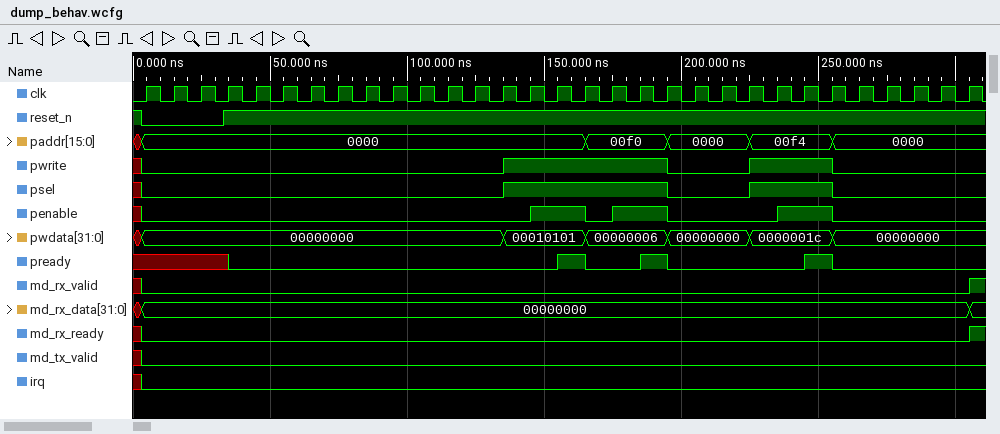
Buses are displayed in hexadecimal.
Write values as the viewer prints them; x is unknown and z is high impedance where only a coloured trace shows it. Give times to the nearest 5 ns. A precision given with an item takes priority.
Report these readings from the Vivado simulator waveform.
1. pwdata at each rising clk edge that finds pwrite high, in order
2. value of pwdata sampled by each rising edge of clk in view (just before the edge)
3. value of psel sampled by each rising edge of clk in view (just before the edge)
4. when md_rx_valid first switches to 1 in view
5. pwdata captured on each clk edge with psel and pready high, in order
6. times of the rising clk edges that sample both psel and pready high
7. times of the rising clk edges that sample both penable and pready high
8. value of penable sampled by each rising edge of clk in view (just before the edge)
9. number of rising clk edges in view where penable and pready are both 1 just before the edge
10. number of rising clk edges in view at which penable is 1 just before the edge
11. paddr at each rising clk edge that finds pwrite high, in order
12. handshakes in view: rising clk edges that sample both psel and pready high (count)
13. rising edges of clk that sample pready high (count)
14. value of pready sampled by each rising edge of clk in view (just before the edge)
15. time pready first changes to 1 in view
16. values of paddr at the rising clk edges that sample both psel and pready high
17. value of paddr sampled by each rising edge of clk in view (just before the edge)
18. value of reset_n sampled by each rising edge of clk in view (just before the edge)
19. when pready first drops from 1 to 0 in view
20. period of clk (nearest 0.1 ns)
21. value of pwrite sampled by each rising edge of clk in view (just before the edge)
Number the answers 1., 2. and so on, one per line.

1. 00010101, 00010101, 00010101, 00000006, 00000006, 00000006, 0000001c, 0000001c, 0000001c
2. 00000000, 00000000, 00000000, 00000000, 00000000, 00000000, 00000000, 00000000, 00000000, 00000000, 00000000, 00000000, 00000000, 00000000, 00010101, 00010101, 00010101, 00000006, 00000006, 00000006, 00000000, 00000000, 00000000, 0000001c, 0000001c, 0000001c, 00000000, 00000000, 00000000, 00000000, 00000000
3. 0 0 0 0 0 0 0 0 0 0 0 0 0 0 1 1 1 1 1 1 0 0 0 1 1 1 0 0 0 0 0
4. 305 ns
5. 00010101, 00000006, 0000001c
6. 165 ns, 195 ns, 255 ns
7. 165 ns, 195 ns, 255 ns
8. 0 0 0 0 0 0 0 0 0 0 0 0 0 0 0 1 1 0 1 1 0 0 0 0 1 1 0 0 0 0 0
9. 3
10. 6
11. 0000, 0000, 0000, 00f0, 00f0, 00f0, 00f4, 00f4, 00f4
12. 3
13. 3
14. x x x x 0 0 0 0 0 0 0 0 0 0 0 0 1 0 0 1 0 0 0 0 0 1 0 0 0 0 0
15. 155 ns
16. 0000, 00f0, 00f4
17. 0000, 0000, 0000, 0000, 0000, 0000, 0000, 0000, 0000, 0000, 0000, 0000, 0000, 0000, 0000, 0000, 0000, 00f0, 00f0, 00f0, 0000, 0000, 0000, 00f4, 00f4, 00f4, 0000, 0000, 0000, 0000, 0000
18. 0 0 0 1 1 1 1 1 1 1 1 1 1 1 1 1 1 1 1 1 1 1 1 1 1 1 1 1 1 1 1
19. 165 ns
20. 10 ns
21. 0 0 0 0 0 0 0 0 0 0 0 0 0 0 1 1 1 1 1 1 0 0 0 1 1 1 0 0 0 0 0
